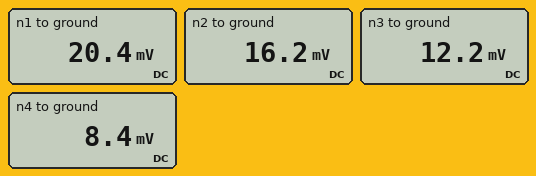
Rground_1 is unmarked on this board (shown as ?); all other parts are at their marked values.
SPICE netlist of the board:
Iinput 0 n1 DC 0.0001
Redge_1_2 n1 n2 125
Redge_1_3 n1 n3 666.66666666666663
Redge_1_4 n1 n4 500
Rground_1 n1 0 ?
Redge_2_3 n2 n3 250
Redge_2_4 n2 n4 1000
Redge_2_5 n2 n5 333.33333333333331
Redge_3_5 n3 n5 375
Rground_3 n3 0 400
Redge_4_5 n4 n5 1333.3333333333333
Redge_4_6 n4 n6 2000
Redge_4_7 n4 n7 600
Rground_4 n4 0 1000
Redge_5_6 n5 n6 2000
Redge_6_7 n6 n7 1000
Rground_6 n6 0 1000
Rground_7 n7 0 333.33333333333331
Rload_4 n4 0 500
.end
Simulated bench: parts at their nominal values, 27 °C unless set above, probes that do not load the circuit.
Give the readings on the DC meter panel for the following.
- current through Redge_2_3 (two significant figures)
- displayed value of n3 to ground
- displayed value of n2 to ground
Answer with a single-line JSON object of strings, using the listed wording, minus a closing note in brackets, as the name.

{"current through Redge_2_3": "16 µA", "displayed value of n3 to ground": "12.2 mV", "displayed value of n2 to ground": "16.2 mV"}
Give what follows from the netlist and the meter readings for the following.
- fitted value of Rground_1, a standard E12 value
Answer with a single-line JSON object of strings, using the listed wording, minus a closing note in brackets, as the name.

{"fitted value of Rground_1, a standard E12 value": "680 Ω"}
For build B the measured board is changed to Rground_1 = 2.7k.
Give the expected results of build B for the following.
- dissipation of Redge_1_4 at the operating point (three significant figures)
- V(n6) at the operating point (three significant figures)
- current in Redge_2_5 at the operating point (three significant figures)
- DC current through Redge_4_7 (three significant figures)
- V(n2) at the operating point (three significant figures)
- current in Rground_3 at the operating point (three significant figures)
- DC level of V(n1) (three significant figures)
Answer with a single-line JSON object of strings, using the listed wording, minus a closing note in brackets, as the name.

{"dissipation of Redge_1_4 at the operating point": "482 nW", "V(n6) at the operating point": "5.99 mV", "current in Redge_2_5 at the operating point": "12.5 µA", "DC current through Redge_4_7": "10.9 µA", "V(n2) at the operating point": "20.9 mV", "current in Rground_3 at the operating point": "39.3 µA", "DC level of V(n1)": "26.3 mV"}
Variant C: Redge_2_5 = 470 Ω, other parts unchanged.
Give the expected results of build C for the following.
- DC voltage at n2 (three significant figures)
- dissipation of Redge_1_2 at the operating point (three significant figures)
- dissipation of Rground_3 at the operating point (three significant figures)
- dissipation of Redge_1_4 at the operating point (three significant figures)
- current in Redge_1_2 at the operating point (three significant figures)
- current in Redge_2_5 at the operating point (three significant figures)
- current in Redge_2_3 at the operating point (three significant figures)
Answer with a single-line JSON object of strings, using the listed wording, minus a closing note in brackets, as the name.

{"DC voltage at n2": "16.4 mV", "dissipation of Redge_1_2 at the operating point": "136 nW", "dissipation of Rground_3 at the operating point": "370 nW", "dissipation of Redge_1_4 at the operating point": "295 nW", "current in Redge_1_2 at the operating point": "33.0 µA", "current in Redge_2_5 at the operating point": "8.15 µA", "current in Redge_2_3 at the operating point": "16.9 µA"}
